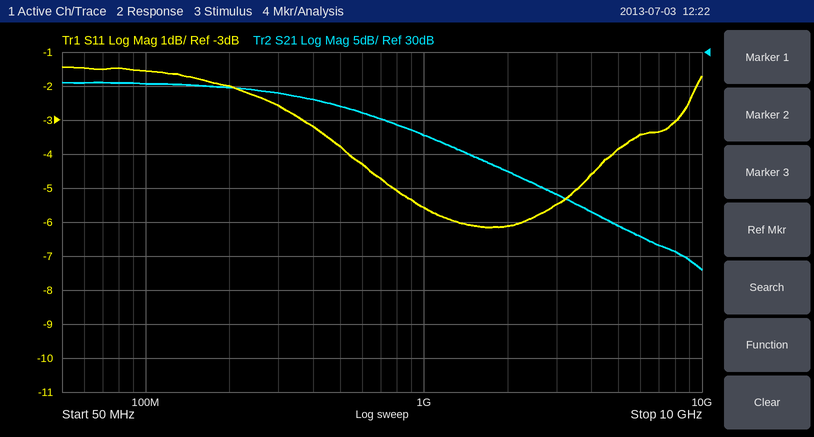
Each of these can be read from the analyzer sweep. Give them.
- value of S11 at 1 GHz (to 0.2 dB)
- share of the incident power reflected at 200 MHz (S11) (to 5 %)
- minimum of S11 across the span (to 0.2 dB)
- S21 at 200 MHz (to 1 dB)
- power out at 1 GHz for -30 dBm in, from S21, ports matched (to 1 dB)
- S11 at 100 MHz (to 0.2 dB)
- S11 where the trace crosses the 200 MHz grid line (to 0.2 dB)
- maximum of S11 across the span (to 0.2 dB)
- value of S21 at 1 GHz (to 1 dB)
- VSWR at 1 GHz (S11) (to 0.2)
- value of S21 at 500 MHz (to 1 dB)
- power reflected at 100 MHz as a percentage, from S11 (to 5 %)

-5.6 dB
65 %
-6.2 dB
25 dB
-12 dBm
-1.6 dB
-2.0 dB
-1.4 dB
18 dB
3.2
22 dB
70 %
